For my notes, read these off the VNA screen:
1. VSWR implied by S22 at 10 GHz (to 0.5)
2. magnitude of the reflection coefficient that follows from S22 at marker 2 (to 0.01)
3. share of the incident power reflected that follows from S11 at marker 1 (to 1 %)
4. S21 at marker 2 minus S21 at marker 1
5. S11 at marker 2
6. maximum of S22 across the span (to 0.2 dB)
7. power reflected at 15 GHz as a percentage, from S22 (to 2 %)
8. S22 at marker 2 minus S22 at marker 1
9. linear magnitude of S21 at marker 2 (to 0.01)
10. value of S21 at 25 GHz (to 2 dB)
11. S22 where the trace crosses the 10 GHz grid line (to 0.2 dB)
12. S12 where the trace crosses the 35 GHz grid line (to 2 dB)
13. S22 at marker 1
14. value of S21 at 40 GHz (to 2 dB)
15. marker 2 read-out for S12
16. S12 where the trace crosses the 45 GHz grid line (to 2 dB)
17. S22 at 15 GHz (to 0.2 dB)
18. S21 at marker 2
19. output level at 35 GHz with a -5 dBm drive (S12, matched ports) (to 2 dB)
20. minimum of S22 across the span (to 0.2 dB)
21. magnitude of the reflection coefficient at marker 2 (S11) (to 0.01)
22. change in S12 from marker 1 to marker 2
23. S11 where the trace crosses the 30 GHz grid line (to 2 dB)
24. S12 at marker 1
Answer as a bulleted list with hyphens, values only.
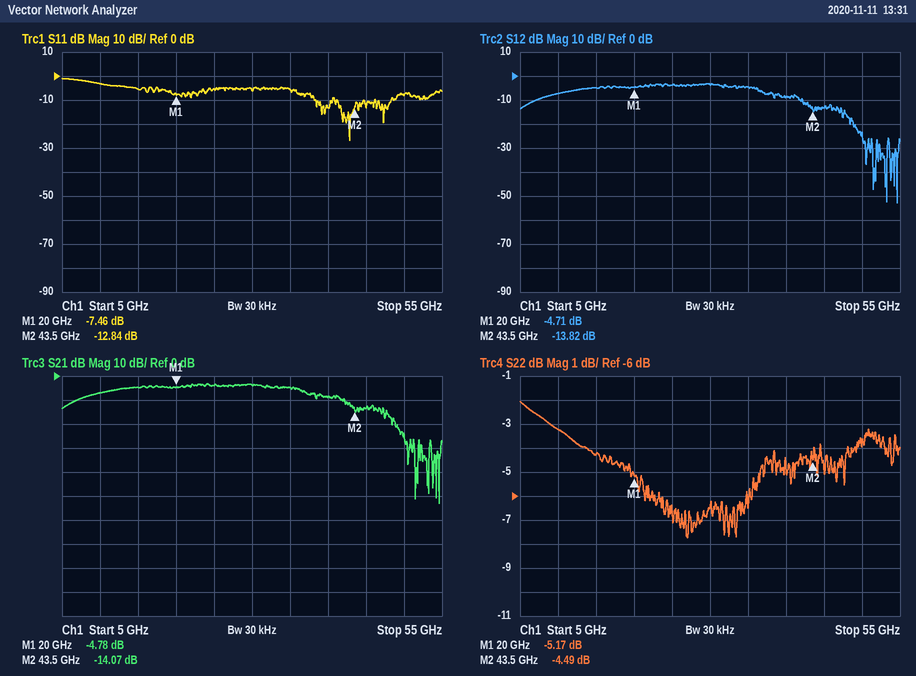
- 5.5
- 0.60
- 18 %
- -9.29 dB
- -12.84 dB
- -2.0 dB
- 38 %
- 0.68 dB
- 0.20
- -4 dB
- -3.2 dB
- -4 dB
- -5.17 dB
- -8 dB
- -13.82 dB
- -14 dB
- -4.2 dB
- -14.07 dB
- -10 dBm
- -7.8 dB
- 0.23
- -9.11 dB
- -6 dB
- -4.71 dB
